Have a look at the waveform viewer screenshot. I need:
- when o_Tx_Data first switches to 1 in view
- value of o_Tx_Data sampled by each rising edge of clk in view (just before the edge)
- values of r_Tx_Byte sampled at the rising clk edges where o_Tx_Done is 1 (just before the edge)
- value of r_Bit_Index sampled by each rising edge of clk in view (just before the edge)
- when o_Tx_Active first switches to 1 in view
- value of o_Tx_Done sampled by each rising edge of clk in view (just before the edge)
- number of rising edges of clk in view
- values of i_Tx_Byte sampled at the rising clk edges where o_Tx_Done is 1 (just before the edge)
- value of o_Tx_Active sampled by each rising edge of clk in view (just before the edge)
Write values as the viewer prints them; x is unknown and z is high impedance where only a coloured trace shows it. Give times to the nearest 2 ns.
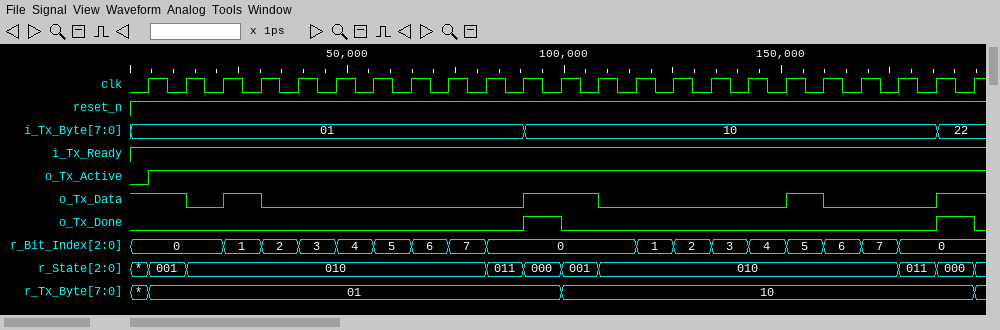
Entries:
22 ns
1 1 0 1 0 0 0 0 0 0 0 1 1 0 0 0 0 0 1 0 0 0 1
01, 10
0, 0, 0, 1, 2, 3, 4, 5, 6, 7, 0, 0, 0, 0, 1, 2, 3, 4, 5, 6, 7, 0, 0
4 ns
0 0 0 0 0 0 0 0 0 0 0 1 0 0 0 0 0 0 0 0 0 0 1
23
10, 22
0 1 1 1 1 1 1 1 1 1 1 1 1 1 1 1 1 1 1 1 1 1 1
